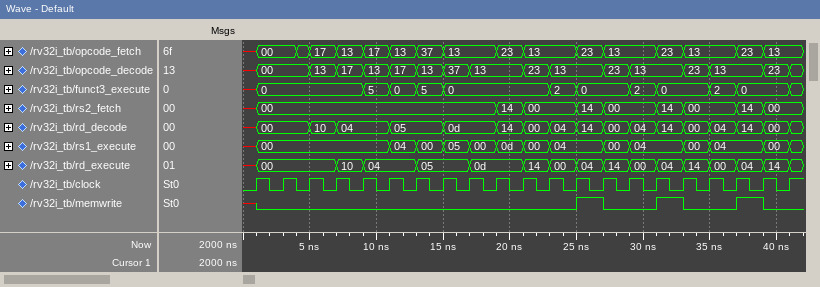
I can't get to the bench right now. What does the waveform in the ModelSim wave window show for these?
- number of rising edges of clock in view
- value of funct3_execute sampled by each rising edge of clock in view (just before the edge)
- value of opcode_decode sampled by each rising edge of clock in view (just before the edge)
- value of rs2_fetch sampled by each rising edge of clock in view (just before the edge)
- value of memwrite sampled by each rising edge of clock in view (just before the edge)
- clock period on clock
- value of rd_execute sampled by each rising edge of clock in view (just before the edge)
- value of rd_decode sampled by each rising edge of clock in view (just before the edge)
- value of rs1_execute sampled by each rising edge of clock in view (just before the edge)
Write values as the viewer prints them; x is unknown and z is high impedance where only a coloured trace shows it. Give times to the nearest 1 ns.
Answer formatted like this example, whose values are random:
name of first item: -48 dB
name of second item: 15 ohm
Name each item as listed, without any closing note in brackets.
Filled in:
number of rising edges of clock in view: 21
value of funct3_execute sampled by each rising edge of clock in view: x, 0, 0, 0, 0, 5, 0, 5, 0, 0, 0, 0, 2, 0, 0, 2, 0, 0, 2, 0, 0
value of opcode_decode sampled by each rising edge of clock in view: x, 00, 00, 13, 17, 13, 17, 13, 37, 13, 13, 23, 13, 13, 23, 13, 13, 23, 13, 13, 23
value of rs2_fetch sampled by each rising edge of clock in view: x, 00, 00, 00, 00, 00, 00, 00, 00, 00, 14, 00, 00, 14, 00, 00, 14, 00, 00, 14, 00
value of memwrite sampled by each rising edge of clock in view: x 0 0 0 0 0 0 0 0 0 0 0 0 1 0 0 1 0 0 1 0
clock period on clock: 2 ns
value of rd_execute sampled by each rising edge of clock in view: x, 00, 00, 00, 10, 04, 04, 05, 05, 0d, 0d, 14, 00, 04, 14, 00, 04, 14, 00, 04, 14
value of rd_decode sampled by each rising edge of clock in view: x, 00, 00, 10, 04, 04, 05, 05, 0d, 0d, 14, 00, 04, 14, 00, 04, 14, 00, 04, 14, 00
value of rs1_execute sampled by each rising edge of clock in view: x, 00, 00, 00, 00, 00, 04, 00, 05, 00, 0d, 00, 04, 04, 00, 04, 04, 00, 04, 04, 00
